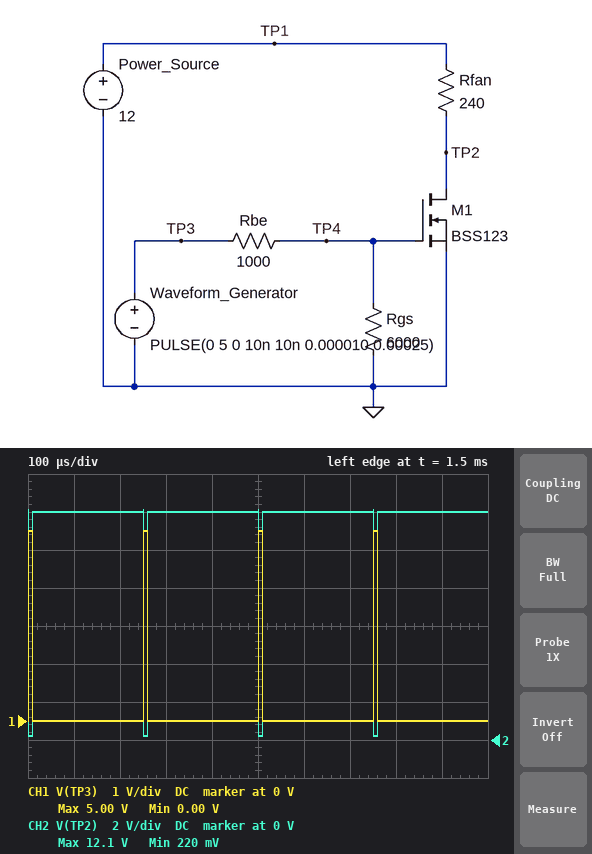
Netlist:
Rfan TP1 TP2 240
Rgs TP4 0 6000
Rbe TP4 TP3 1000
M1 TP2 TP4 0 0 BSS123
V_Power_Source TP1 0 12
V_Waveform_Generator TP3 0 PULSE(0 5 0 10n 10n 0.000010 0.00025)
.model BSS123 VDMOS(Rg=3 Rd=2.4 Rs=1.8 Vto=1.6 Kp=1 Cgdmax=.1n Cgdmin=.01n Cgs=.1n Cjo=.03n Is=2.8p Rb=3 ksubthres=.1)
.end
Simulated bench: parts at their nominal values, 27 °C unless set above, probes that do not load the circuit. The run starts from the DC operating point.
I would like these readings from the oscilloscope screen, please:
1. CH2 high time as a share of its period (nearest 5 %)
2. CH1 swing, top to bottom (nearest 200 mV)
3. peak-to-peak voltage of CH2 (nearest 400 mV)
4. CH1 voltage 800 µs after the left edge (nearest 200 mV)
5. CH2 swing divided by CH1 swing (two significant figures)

95 %
5.0 V
12.0 V
0 V
2.4
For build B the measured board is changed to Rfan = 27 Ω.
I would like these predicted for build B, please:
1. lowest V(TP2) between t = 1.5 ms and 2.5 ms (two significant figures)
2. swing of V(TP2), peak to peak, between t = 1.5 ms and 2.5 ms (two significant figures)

1.8 V
10 V
